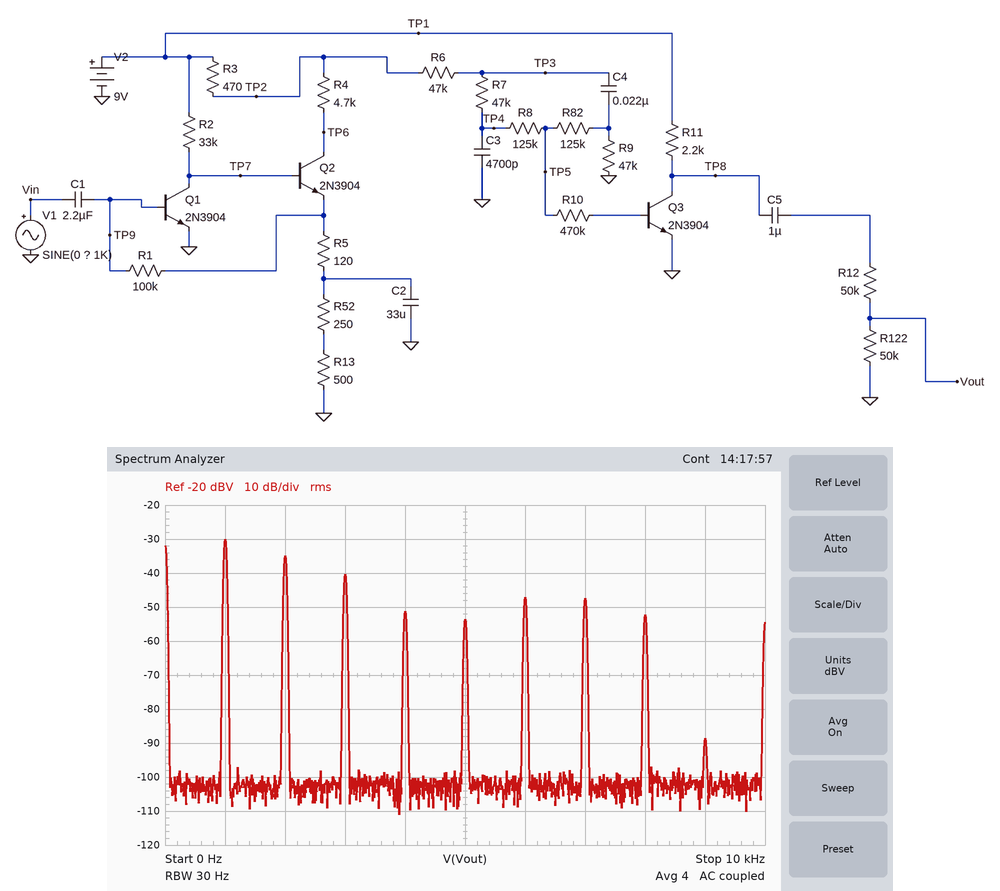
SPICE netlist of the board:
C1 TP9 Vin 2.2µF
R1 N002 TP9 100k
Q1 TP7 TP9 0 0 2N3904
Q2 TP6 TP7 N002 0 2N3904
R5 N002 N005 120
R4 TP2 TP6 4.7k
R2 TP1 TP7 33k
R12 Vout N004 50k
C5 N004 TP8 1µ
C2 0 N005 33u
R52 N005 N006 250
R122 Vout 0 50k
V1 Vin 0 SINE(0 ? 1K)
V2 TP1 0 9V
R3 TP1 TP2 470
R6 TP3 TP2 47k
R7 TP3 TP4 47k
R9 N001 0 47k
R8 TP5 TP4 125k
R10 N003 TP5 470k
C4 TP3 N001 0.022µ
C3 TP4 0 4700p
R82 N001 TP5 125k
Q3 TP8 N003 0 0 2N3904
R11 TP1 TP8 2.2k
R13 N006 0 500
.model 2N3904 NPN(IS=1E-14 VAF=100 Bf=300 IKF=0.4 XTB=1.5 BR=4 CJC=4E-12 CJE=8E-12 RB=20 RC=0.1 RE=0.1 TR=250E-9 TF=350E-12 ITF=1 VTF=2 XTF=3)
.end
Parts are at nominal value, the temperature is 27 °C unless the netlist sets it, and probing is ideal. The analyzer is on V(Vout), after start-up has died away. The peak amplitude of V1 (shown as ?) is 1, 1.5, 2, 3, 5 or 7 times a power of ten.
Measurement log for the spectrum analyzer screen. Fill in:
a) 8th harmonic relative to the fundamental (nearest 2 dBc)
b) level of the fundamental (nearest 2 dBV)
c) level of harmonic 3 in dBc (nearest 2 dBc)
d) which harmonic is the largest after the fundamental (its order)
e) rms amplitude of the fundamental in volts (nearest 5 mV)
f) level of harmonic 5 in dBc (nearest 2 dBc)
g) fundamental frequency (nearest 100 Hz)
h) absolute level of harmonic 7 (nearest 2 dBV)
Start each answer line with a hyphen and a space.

- -22 dBc
- -30 dBV
- -10 dBc
- 2
- 30 mV
- -24 dBc
- 1.0 kHz
- -48 dBV
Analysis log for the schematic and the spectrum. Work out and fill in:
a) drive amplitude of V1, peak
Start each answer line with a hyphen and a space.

- 100 mV
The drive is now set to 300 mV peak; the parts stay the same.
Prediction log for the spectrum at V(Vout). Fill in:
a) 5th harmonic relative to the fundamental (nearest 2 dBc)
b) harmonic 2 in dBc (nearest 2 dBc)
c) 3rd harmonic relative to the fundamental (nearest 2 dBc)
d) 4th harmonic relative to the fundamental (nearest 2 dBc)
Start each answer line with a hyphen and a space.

- -16 dBc
- -4 dBc
- -6 dBc
- -10 dBc
